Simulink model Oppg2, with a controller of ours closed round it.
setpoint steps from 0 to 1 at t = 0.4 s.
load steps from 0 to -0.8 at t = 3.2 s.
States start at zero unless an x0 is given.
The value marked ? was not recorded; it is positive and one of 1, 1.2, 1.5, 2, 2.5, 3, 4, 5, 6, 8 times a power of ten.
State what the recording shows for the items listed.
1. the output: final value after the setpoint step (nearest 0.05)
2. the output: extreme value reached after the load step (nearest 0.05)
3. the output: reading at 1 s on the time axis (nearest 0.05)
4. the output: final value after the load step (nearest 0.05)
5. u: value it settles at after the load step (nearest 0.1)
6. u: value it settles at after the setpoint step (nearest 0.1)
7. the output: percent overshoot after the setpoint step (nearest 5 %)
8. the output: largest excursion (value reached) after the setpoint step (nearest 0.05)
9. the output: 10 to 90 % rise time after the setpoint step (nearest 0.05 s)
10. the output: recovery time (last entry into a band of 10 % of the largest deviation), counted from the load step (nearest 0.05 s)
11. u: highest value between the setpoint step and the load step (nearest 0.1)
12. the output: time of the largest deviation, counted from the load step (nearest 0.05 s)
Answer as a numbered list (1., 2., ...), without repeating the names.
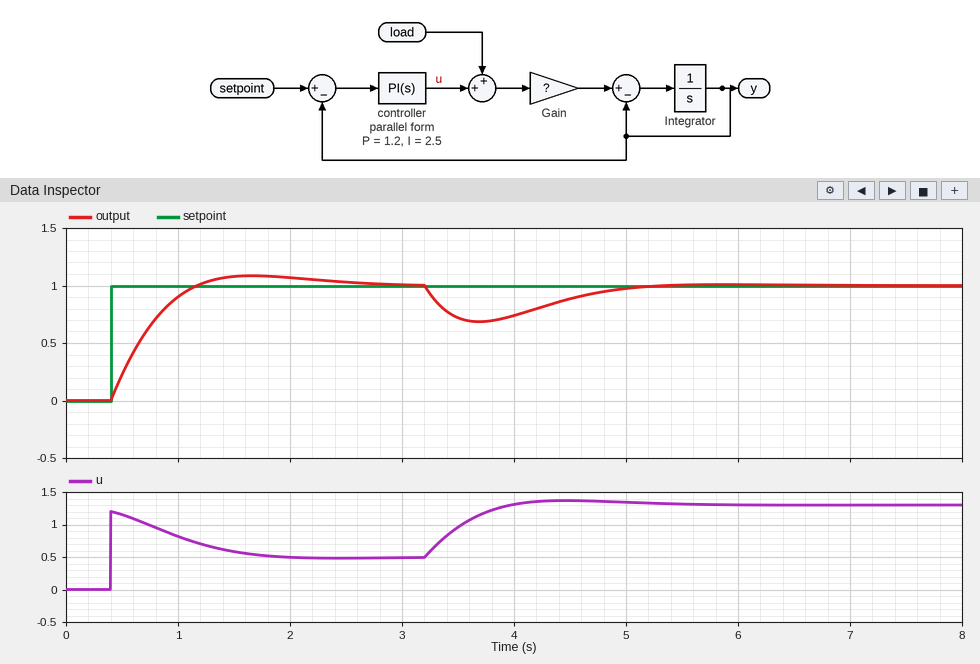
1. 1.00
2. 0.70
3. 0.90
4. 1.00
5. 1.3
6. 0.5
7. 10 %
8. 1.10
9. 0.55 s
10. 1.75 s
11. 1.2
12. 0.50 s
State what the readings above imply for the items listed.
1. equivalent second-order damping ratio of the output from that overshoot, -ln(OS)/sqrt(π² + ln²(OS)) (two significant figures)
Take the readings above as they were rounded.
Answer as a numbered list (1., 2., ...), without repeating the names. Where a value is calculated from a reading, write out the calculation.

1. ln(0.1) = -2.303; 2.303 / sqrt(9.870 + 5.302) = 0.59
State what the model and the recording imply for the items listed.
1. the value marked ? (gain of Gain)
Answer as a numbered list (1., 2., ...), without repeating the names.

1. 2
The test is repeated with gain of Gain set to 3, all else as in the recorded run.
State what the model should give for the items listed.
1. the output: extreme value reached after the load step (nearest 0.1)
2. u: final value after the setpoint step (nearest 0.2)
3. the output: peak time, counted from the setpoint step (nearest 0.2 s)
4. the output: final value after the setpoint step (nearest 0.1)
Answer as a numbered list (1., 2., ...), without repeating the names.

1. 0.6
2. 0.4
3. 1.0 s
4. 1.0
